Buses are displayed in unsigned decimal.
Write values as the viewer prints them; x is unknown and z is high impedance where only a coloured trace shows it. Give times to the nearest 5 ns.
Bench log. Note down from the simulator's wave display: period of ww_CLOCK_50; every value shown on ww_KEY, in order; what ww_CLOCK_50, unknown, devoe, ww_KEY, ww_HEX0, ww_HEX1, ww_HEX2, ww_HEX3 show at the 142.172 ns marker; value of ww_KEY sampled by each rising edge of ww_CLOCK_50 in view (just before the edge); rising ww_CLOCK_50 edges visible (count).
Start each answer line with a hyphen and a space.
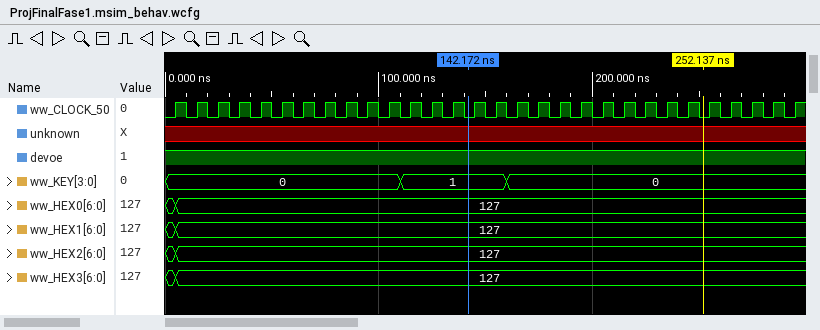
- 10 ns
- 0, 1, 0
- ww_CLOCK_50=0, unknown=x, devoe=1, ww_KEY=1, ww_HEX0=127, ww_HEX1=127, ww_HEX2=127, ww_HEX3=127
- 0, 0, 0, 0, 0, 0, 0, 0, 0, 0, 0, 1, 1, 1, 1, 1, 0, 0, 0, 0, 0, 0, 0, 0, 0, 0, 0, 0, 0, 0
- 30
